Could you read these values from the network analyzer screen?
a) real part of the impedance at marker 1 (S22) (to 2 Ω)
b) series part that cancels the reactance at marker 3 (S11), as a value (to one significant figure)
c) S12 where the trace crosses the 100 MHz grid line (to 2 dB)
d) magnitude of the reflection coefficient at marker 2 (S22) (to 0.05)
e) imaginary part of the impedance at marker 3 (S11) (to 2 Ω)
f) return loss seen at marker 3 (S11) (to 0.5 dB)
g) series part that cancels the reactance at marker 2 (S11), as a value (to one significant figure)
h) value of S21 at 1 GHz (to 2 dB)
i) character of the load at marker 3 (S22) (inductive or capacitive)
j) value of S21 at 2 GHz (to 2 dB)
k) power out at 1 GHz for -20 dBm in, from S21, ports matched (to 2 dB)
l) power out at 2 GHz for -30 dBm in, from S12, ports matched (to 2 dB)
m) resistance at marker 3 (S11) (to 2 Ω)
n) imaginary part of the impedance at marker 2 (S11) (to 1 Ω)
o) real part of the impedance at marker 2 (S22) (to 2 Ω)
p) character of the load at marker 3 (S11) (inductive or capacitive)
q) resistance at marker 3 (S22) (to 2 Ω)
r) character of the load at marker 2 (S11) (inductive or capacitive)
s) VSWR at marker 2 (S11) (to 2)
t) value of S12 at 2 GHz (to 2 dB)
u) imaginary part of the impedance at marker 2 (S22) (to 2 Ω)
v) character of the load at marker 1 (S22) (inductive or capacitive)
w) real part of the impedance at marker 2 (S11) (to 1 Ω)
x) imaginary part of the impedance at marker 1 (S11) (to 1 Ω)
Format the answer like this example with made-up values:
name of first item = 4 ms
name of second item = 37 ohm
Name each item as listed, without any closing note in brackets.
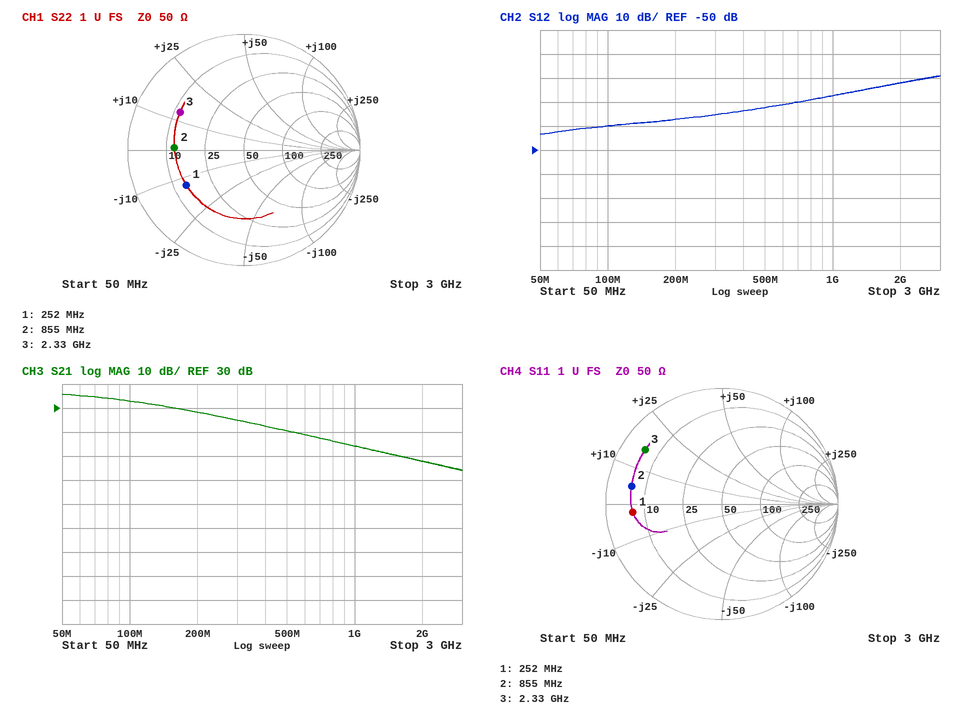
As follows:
real part of the impedance at marker 1 (S22) = 14 Ω
series part that cancels the reactance at marker 3 (S11), as a value = 4 pF
S12 where the trace crosses the 100 MHz grid line = -40 dB
magnitude of the reflection coefficient at marker 2 (S22) = 0.60
imaginary part of the impedance at marker 3 (S11) = +16 Ω
return loss seen at marker 3 (S11) = 2.0 dB
series part that cancels the reactance at marker 2 (S11), as a value = 40 pF
value of S21 at 1 GHz = 14 dB
character of the load at marker 3 (S22) = inductive
value of S21 at 2 GHz = 8 dB
power out at 1 GHz for -20 dBm in, from S21, ports matched = -6 dBm
power out at 2 GHz for -30 dBm in, from S12, ports matched = -52 dBm
resistance at marker 3 (S11) = 6 Ω
imaginary part of the impedance at marker 2 (S11) = +5 Ω
real part of the impedance at marker 2 (S22) = 12 Ω
character of the load at marker 3 (S11) = inductive
resistance at marker 3 (S22) = 12 Ω
character of the load at marker 2 (S11) = inductive
VSWR at marker 2 (S11) = 8
value of S12 at 2 GHz = -22 dB
imaginary part of the impedance at marker 2 (S22) = 0 Ω
character of the load at marker 1 (S22) = capacitive
real part of the impedance at marker 2 (S11) = 6 Ω
imaginary part of the impedance at marker 1 (S11) = -2 Ω
